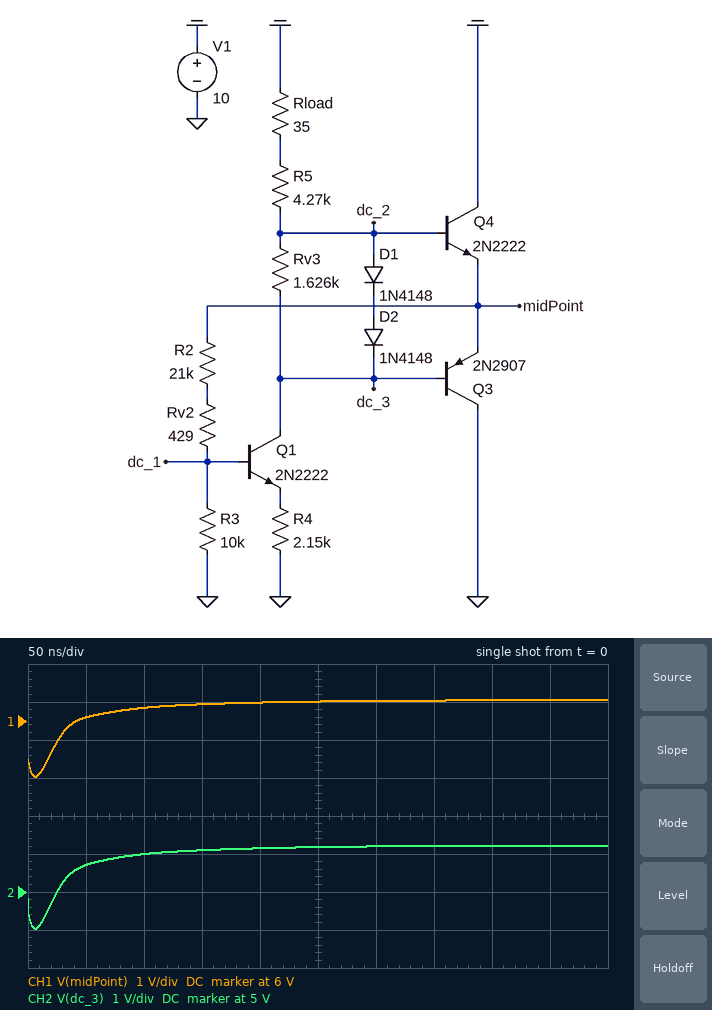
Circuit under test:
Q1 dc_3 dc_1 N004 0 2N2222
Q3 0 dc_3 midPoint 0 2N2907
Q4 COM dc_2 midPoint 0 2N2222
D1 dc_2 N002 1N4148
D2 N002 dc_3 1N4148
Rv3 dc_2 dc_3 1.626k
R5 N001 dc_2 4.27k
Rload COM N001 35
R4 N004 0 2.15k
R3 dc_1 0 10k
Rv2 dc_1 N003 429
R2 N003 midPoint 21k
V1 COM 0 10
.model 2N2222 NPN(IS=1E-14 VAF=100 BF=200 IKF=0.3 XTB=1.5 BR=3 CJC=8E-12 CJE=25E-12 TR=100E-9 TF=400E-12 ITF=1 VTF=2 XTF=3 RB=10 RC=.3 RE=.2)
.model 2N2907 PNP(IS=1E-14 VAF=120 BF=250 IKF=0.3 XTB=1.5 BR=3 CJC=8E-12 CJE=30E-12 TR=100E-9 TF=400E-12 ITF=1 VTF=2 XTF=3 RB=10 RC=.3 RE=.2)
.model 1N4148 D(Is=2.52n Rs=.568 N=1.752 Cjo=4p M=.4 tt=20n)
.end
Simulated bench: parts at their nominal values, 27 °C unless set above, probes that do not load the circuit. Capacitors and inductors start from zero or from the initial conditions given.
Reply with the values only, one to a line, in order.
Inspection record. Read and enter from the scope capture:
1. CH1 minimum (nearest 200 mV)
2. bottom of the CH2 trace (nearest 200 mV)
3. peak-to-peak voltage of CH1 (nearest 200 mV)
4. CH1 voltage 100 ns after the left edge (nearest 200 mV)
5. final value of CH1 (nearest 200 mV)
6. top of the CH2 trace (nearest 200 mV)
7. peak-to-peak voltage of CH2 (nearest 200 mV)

4.6 V
4.0 V
2.0 V
6.4 V
6.6 V
6.2 V
2.2 V
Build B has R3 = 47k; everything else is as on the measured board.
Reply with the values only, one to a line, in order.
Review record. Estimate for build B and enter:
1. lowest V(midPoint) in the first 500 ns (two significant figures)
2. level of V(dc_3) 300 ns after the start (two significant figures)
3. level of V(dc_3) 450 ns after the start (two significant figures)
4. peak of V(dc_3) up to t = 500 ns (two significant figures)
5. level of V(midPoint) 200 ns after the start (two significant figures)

4.6 V
4.3 V
4.1 V
5.3 V
5.0 V
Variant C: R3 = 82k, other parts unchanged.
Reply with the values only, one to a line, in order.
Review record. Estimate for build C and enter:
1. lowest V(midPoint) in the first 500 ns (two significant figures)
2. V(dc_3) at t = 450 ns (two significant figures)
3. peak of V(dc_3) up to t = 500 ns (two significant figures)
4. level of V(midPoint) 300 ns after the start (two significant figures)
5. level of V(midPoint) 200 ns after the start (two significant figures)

4.3 V
3.8 V
5.3 V
4.5 V
4.7 V
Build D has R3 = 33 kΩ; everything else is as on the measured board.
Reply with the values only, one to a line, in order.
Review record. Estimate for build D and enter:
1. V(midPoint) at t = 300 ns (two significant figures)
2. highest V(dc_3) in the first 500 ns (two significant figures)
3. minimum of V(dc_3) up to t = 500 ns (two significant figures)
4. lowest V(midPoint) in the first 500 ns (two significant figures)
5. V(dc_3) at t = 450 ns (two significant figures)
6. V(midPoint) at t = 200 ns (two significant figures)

5.0 V
5.4 V
4.1 V
4.6 V
4.5 V
5.2 V
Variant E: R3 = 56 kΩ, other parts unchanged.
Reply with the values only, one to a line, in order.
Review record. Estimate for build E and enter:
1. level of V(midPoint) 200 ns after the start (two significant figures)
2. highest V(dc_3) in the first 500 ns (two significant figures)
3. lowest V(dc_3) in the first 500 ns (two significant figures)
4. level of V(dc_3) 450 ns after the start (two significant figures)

4.9 V
5.3 V
4.0 V
4.0 V
